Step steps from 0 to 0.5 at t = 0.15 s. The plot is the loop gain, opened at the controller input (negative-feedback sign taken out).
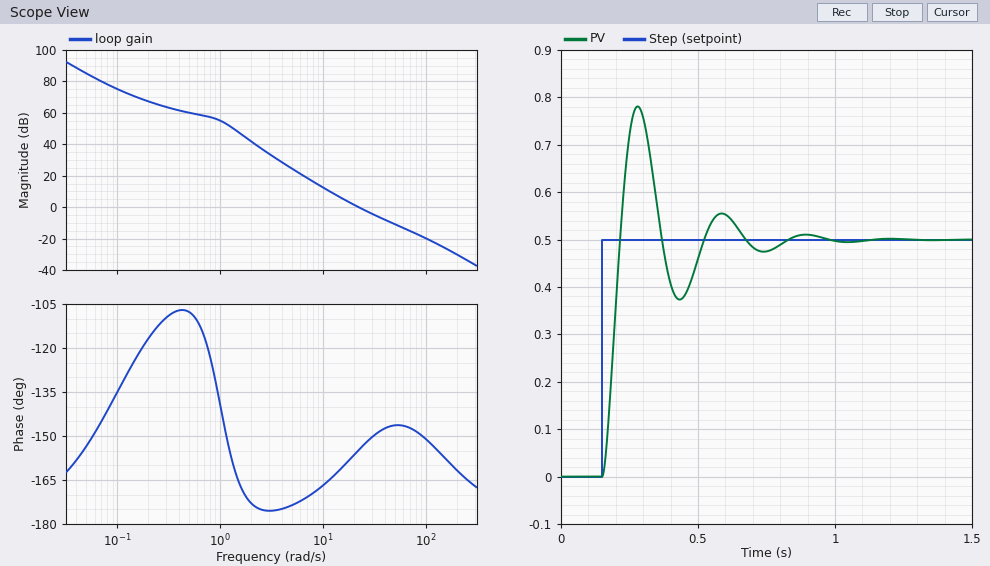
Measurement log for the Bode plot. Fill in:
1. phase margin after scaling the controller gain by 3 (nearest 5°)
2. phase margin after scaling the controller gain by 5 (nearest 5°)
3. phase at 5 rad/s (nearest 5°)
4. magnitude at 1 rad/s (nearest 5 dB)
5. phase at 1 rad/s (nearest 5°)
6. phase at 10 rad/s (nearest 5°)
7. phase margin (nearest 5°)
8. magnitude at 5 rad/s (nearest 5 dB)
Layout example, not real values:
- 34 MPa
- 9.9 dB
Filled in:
- 35°
- 35°
- -175°
- 55 dB
- -140°
- -165°
- 25°
- 25 dB
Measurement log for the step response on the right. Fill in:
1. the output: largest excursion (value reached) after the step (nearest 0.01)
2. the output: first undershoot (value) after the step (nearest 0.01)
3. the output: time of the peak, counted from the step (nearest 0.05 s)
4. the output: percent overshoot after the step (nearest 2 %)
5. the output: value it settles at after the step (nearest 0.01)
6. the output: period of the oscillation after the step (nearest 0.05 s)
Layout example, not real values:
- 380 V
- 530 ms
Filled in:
- 0.78
- 0.37
- 0.15 s
- 56 %
- 0.50
- 0.30 s
